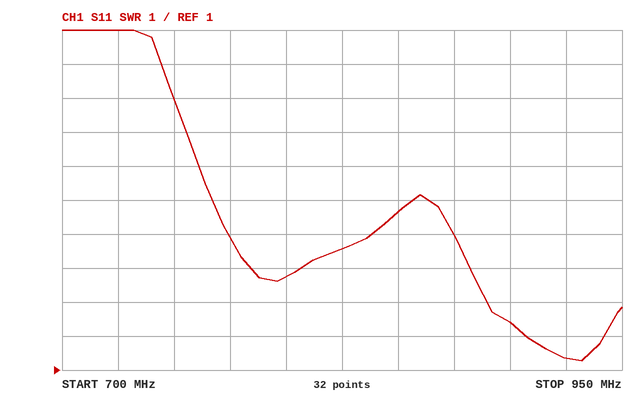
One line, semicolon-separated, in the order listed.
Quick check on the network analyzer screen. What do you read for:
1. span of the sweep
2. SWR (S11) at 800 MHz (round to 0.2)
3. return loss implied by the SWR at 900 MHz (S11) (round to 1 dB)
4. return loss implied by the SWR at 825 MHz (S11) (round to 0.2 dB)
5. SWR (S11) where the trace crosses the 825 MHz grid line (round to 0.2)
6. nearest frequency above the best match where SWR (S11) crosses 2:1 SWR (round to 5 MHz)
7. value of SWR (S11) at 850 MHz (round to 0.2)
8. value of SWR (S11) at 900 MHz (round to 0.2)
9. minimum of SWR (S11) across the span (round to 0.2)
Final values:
250 MHz; 3.8; 8 dB; 3.8 dB; 4.6; 940 MHz; 5.6; 2.4; 1.2
